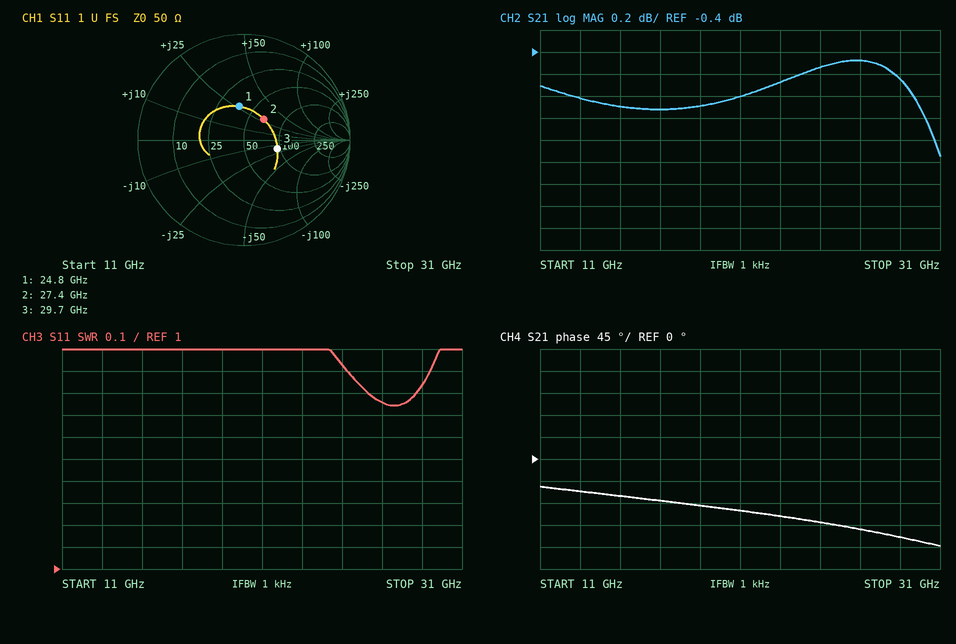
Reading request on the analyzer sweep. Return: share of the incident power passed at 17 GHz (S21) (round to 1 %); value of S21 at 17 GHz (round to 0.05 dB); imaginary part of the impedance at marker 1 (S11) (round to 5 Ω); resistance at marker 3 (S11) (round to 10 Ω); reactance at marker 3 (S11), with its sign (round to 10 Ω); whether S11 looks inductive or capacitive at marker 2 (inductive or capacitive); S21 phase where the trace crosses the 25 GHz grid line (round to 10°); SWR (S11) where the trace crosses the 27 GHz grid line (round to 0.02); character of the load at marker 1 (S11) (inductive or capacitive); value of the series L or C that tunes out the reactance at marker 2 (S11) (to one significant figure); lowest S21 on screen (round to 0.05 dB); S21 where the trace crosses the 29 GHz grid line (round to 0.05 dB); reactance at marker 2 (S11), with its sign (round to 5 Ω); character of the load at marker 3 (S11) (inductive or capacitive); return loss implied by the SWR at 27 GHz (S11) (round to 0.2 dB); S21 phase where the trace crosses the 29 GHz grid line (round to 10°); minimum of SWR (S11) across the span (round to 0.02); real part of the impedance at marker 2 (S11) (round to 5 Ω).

81 %
-0.90 dB
+25 Ω
90 Ω
-20 Ω
inductive
-130°
1.76
inductive
200 fF
-1.35 dB
-0.65 dB
+30 Ω
capacitive
11.2 dB
-160°
1.74
65 Ω
